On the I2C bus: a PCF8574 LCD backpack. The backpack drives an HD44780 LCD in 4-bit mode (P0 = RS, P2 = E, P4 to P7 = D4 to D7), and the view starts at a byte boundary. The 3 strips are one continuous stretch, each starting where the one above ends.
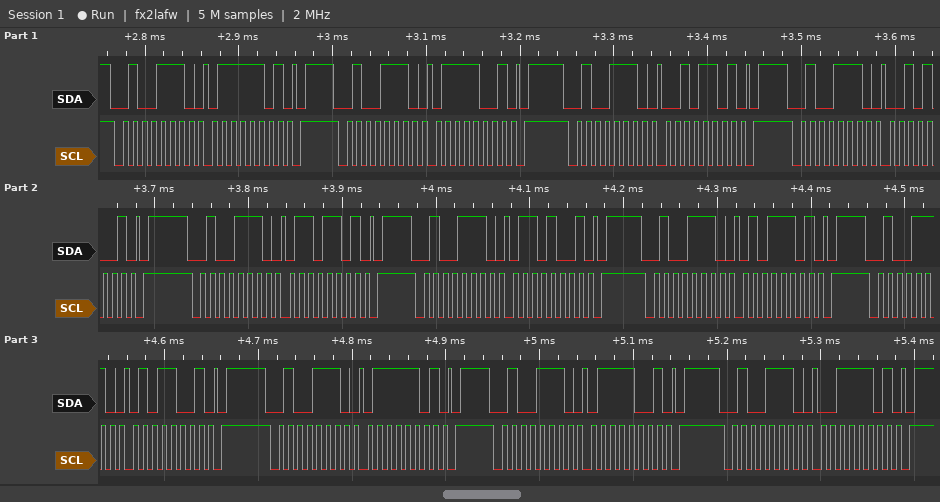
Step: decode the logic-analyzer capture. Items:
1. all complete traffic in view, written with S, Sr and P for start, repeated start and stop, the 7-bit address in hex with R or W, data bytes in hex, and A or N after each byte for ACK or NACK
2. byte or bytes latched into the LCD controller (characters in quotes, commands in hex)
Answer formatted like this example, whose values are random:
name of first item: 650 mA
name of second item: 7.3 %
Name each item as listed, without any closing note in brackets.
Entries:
all complete traffic in view, written with S, Sr and P for start, repeated start and stop, the 7-bit address in hex with R or W, data bytes in hex, and A or N after each byte for ACK or NACK: S 27W A 7D A P S 27W A 79 A P S 27W A 2D A P S 27W A 29 A P S 27W A 6D A P S 27W A 69 A P S 27W A 5D A P S 27W A 59 A P S 27W A 7D A P S 27W A 79 A P S 27W A 3D A P
byte or bytes latched into the LCD controller: 'r' 'e'
